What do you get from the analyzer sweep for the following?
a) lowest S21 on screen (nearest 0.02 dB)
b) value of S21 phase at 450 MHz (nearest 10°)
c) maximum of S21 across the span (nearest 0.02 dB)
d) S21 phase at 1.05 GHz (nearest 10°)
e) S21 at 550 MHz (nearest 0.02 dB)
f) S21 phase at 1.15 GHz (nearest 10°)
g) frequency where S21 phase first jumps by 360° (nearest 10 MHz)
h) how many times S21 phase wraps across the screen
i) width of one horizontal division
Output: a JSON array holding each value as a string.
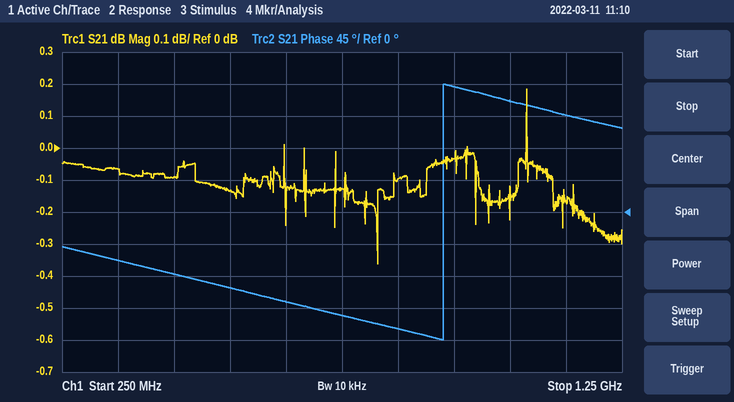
["-0.36 dB", "-90°", "0.18 dB", "160°", "-0.14 dB", "140°", "930 MHz", "1", "100 MHz"]
